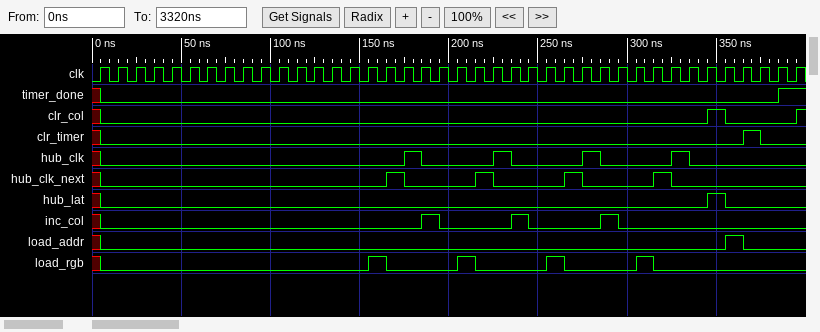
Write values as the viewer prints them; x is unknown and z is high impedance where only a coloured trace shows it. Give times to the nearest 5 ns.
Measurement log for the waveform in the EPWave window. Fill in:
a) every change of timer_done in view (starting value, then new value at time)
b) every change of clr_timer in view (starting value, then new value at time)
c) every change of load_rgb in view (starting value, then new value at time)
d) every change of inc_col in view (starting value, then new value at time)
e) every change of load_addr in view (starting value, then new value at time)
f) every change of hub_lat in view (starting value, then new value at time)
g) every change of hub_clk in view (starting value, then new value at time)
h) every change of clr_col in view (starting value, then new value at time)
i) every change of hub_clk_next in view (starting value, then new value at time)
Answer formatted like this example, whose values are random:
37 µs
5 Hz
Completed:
x, 0 at 5 ns, 1 at 385 ns
x, 0 at 5 ns, 1 at 365 ns, 0 at 375 ns
x, 0 at 5 ns, 1 at 155 ns, 0 at 165 ns, 1 at 205 ns, 0 at 215 ns, 1 at 255 ns, 0 at 265 ns, 1 at 305 ns, 0 at 315 ns
x, 0 at 5 ns, 1 at 185 ns, 0 at 195 ns, 1 at 235 ns, 0 at 245 ns, 1 at 285 ns, 0 at 295 ns
x, 0 at 5 ns, 1 at 355 ns, 0 at 365 ns
x, 0 at 5 ns, 1 at 345 ns, 0 at 355 ns
x, 0 at 5 ns, 1 at 175 ns, 0 at 185 ns, 1 at 225 ns, 0 at 235 ns, 1 at 275 ns, 0 at 285 ns, 1 at 325 ns, 0 at 335 ns
x, 0 at 5 ns, 1 at 345 ns, 0 at 355 ns, 1 at 395 ns
x, 0 at 5 ns, 1 at 165 ns, 0 at 175 ns, 1 at 215 ns, 0 at 225 ns, 1 at 265 ns, 0 at 275 ns, 1 at 315 ns, 0 at 325 ns
